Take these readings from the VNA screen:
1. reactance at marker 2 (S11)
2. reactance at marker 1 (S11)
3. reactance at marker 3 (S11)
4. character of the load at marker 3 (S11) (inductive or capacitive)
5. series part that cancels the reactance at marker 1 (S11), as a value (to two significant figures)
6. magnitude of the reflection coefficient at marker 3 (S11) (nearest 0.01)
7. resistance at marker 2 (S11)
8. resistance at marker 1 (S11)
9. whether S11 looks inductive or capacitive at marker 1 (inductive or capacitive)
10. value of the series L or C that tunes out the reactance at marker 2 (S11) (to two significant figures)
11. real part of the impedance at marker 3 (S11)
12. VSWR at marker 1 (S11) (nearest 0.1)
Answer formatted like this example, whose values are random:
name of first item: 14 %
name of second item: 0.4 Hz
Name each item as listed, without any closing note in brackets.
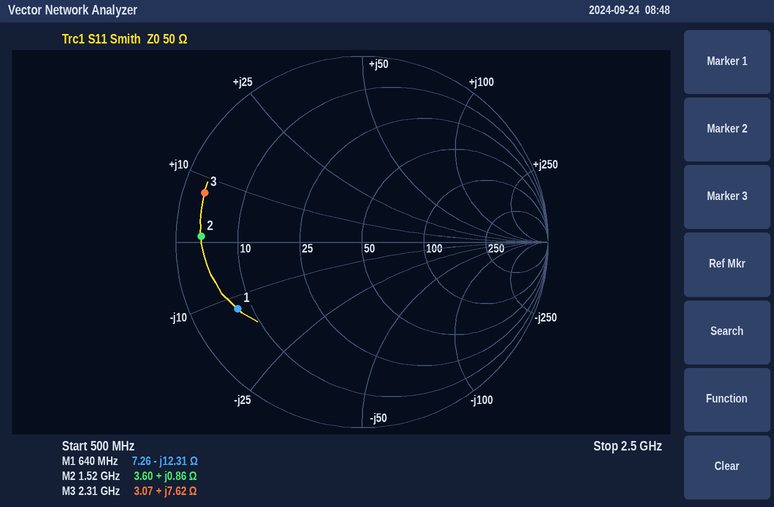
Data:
reactance at marker 2: +0.86 Ω
reactance at marker 1: -12.31 Ω
reactance at marker 3: +7.62 Ω
character of the load at marker 3 (S11): inductive
series part that cancels the reactance at marker 1 (S11), as a value: 3.1 nH
magnitude of the reflection coefficient at marker 3 (S11): 0.89
resistance at marker 2: 3.60 Ω
resistance at marker 1: 7.26 Ω
whether S11 looks inductive or capacitive at marker 1: capacitive
value of the series L or C that tunes out the reactance at marker 2 (S11): 120 pF
real part of the impedance at marker 3: 3.07 Ω
VSWR at marker 1 (S11): 7.3
